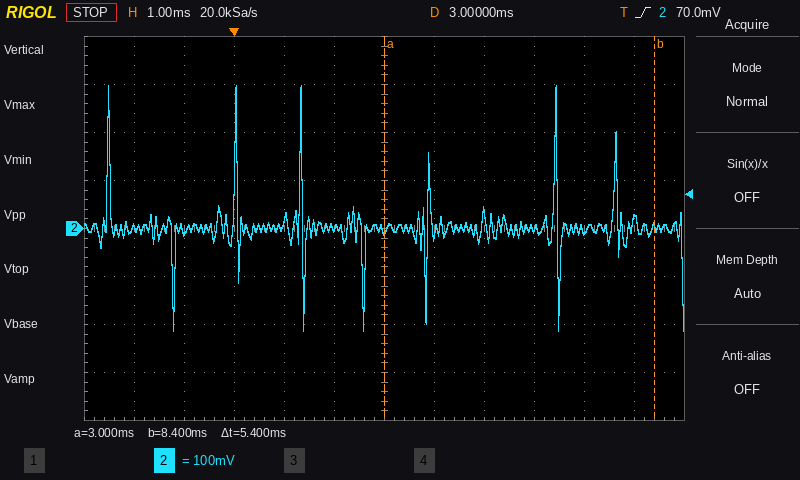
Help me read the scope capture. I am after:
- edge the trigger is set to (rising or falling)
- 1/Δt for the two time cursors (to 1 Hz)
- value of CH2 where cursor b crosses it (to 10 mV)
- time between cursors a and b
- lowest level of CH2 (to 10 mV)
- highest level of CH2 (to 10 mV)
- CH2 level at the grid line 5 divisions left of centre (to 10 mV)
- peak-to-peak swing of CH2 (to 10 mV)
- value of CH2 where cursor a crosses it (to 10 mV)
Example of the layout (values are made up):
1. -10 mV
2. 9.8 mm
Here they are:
1. rising
2. 185 Hz
3. 0 mV
4. 5.4 ms
5. -210 mV
6. 300 mV
7. 0 mV
8. 510 mV
9. 0 mV
